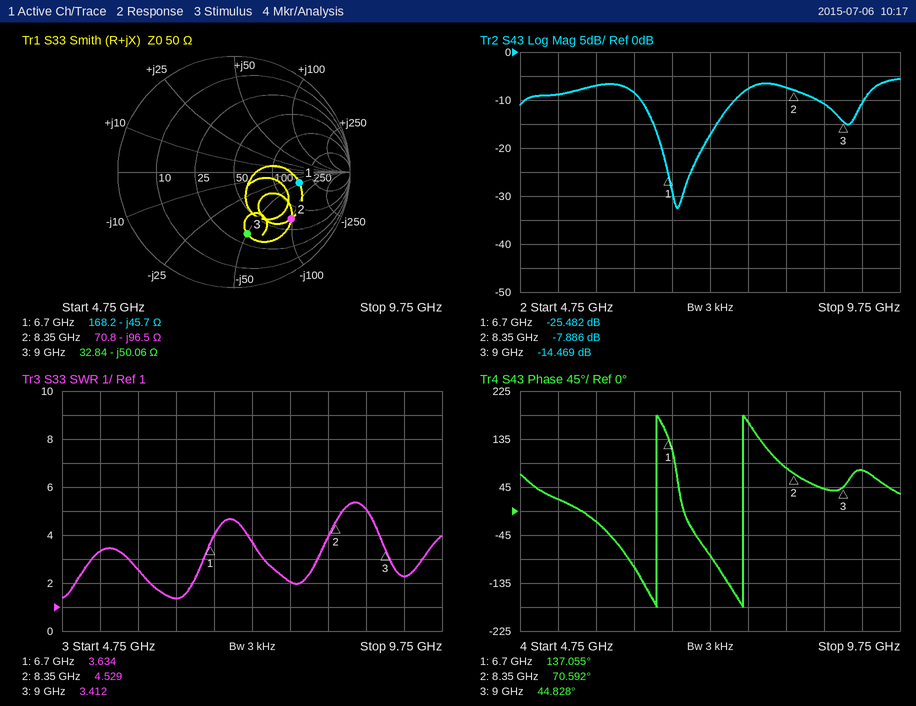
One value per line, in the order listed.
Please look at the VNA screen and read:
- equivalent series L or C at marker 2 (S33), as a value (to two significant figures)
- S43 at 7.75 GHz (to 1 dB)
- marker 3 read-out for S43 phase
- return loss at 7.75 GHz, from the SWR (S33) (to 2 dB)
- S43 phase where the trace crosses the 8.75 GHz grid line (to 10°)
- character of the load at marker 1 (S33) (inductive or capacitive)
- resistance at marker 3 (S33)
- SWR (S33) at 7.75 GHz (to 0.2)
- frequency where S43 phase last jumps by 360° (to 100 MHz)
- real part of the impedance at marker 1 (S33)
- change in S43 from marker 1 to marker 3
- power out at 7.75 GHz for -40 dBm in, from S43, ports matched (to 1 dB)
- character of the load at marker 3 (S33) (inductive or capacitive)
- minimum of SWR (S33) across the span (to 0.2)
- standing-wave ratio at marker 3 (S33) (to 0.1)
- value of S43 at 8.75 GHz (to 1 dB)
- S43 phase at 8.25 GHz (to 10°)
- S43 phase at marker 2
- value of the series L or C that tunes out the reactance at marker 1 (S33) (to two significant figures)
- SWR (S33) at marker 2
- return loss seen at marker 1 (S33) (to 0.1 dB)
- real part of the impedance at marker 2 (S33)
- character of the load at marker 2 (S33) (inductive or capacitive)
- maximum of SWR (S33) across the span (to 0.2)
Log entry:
200 fF
-8 dB
44.828°
10 dB
40°
capacitive
32.84 Ω
2.0
7.7 GHz
168.2 Ω
11.013 dB
-48 dBm
capacitive
1.4
3.4
-11 dB
80°
70.592°
1.1 nH
4.529
4.9 dB
70.8 Ω
capacitive
5.4
